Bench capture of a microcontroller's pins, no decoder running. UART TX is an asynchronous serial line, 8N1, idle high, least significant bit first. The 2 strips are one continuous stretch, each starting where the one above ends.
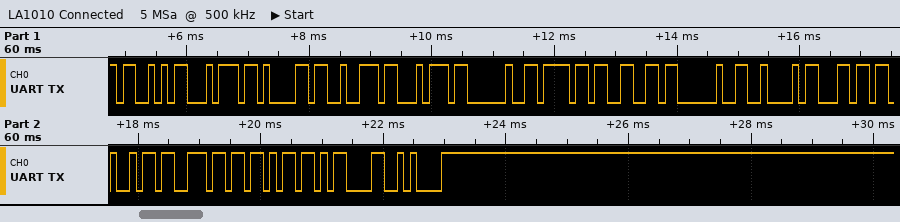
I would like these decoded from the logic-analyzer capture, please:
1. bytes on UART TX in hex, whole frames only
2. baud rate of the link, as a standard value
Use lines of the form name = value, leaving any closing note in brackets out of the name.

bytes on UART TX in hex, whole frames only = 0x53 0x74 0x61 0x72 0x74 0x20 0x6F 0x66 0x20 0x42 0x6C 0x69 0x6E 0x6B 0x0D 0x0A
baud rate of the link, as a standard value = 9600 baud
